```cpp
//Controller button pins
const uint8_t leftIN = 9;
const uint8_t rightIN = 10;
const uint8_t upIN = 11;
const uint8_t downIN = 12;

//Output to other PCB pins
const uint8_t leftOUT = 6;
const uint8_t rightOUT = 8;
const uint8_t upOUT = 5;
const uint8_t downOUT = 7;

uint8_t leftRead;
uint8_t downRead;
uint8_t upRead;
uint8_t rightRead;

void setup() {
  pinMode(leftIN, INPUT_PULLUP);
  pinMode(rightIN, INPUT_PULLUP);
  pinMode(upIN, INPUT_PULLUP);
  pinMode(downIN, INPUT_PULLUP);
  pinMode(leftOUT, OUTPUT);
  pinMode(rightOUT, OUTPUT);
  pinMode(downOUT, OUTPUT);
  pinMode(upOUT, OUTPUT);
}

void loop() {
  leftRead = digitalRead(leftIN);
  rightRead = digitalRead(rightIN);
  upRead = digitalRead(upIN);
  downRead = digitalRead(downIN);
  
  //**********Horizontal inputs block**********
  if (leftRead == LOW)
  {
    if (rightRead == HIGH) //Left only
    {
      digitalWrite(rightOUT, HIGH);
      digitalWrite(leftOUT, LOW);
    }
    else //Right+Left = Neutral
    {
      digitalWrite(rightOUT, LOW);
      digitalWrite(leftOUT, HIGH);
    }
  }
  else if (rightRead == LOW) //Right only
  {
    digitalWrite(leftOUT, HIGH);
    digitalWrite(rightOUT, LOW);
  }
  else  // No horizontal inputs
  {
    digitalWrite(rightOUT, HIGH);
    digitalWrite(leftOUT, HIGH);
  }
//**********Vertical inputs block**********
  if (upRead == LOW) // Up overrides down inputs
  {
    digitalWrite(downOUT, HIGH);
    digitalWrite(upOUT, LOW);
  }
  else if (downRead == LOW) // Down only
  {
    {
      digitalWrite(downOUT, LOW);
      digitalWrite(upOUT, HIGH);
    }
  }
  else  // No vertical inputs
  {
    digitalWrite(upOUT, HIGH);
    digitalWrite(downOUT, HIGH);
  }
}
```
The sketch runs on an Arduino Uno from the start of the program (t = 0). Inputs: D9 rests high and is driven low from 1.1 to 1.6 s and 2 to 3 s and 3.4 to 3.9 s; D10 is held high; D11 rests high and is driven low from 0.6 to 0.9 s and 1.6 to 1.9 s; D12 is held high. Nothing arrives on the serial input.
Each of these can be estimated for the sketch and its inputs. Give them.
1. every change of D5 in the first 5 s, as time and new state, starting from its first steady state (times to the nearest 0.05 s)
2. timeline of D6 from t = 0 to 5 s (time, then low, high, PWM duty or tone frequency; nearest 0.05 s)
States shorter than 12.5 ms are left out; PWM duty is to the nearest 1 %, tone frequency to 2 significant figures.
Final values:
0 s high; 0.6 s low; 0.9 s high; 1.6 s low; 1.9 s high
0 s high; 1.1 s low; 1.6 s high; 2 s low; 3 s high; 3.4 s low; 3.9 s high
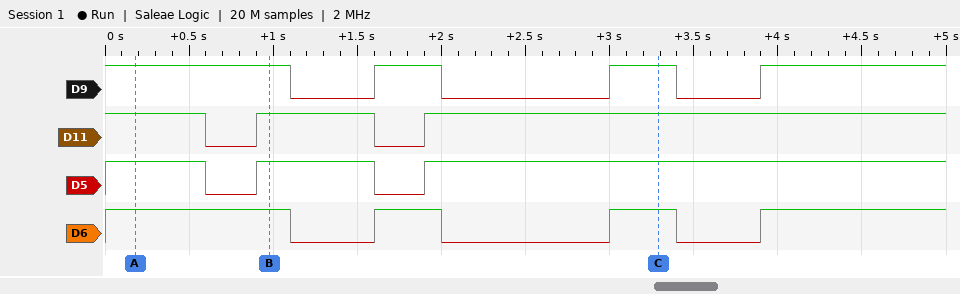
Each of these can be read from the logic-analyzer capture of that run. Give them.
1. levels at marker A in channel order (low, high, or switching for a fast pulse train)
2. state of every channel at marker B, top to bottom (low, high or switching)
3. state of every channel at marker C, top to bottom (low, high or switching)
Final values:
D9 high, D11 high, D5 high, D6 high
D9 high, D11 high, D5 high, D6 high
D9 high, D11 high, D5 high, D6 high
